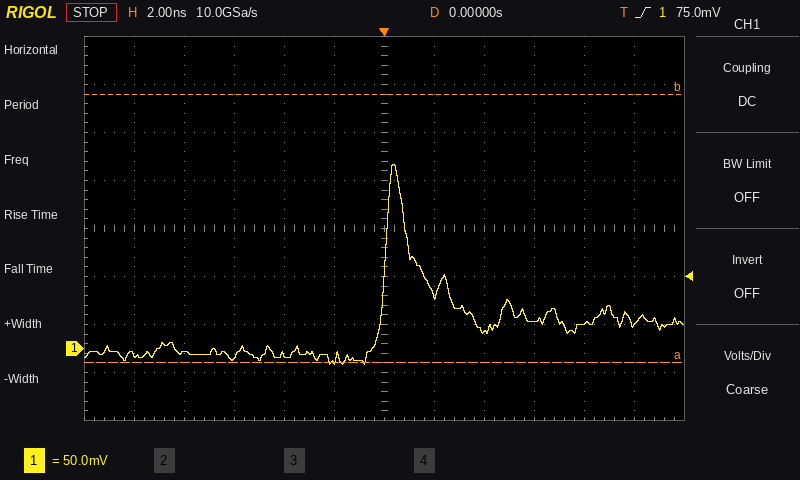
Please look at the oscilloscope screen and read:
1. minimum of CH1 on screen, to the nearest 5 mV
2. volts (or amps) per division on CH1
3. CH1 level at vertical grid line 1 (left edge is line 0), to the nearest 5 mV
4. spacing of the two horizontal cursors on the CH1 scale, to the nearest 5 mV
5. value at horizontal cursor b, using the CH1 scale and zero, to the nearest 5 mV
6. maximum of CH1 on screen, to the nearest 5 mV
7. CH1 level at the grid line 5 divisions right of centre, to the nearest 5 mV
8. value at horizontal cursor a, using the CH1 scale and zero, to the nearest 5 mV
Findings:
-15 mV
50 mV
-5 mV
280 mV
265 mV
190 mV
25 mV
-15 mV
